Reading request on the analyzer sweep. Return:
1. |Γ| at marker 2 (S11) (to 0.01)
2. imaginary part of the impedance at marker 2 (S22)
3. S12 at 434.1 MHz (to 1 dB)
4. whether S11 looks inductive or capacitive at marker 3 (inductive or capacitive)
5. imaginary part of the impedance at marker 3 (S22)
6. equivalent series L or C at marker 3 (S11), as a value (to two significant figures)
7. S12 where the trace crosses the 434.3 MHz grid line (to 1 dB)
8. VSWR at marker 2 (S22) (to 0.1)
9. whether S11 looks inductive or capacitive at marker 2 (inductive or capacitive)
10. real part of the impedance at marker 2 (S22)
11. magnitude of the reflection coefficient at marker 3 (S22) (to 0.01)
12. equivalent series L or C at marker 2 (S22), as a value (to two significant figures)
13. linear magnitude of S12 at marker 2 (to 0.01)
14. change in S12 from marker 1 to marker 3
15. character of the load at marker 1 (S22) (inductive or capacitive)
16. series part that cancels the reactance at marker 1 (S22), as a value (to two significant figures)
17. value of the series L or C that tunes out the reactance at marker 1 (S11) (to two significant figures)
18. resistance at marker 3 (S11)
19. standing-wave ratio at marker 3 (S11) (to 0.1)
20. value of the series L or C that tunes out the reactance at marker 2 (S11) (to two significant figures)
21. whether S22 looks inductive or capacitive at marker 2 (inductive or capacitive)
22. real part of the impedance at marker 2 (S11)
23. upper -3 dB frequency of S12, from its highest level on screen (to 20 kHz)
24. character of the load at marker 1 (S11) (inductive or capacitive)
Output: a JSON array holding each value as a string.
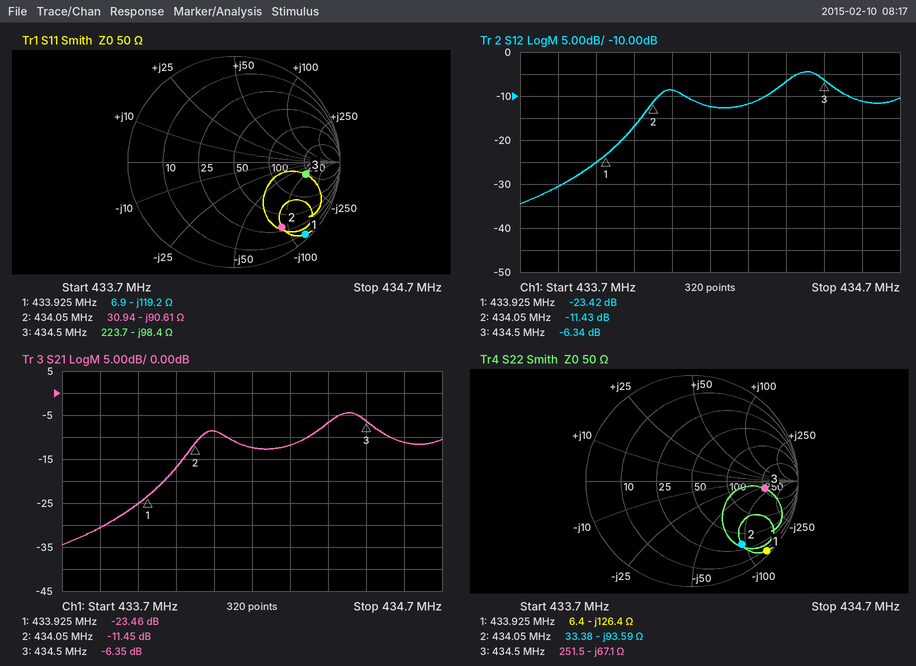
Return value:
["0.76", "-93.59 Ω", "-9 dB", "capacitive", "-67.1 Ω", "3.7 pF", "-12 dB", "7.3", "capacitive", "33.38 Ω", "0.69", "3.9 pF", "0.27", "17.08 dB", "capacitive", "46 nH", "44 nH", "223.7 Ω", "5.4", "33 nH", "capacitive", "30.94 Ω", "434.52 MHz", "capacitive"]
